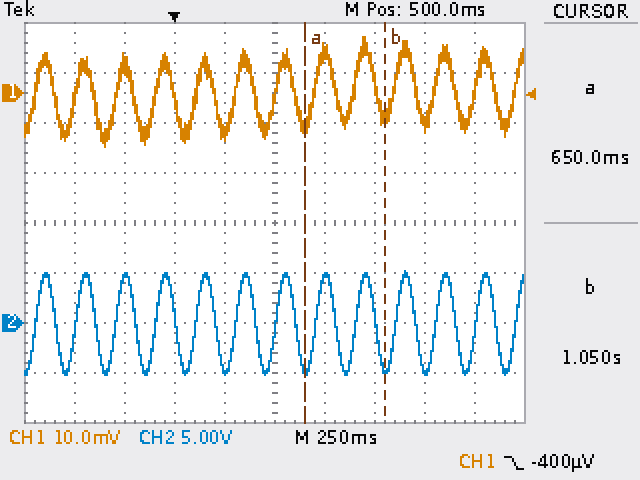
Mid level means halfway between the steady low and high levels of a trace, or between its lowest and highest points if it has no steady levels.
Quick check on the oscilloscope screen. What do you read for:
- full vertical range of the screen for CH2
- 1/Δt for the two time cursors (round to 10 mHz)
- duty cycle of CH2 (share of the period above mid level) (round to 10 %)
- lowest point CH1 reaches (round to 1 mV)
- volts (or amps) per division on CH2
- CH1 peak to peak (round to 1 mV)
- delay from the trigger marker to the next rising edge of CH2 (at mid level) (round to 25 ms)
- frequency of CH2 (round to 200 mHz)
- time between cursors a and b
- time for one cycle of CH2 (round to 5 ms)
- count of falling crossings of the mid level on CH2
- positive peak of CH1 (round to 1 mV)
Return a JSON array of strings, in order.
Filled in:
["40 V", "2.50 Hz", "50 %", "-11 mV", "5 V", "22 mV", "100 ms", "5.0 Hz", "400 ms", "200 ms", "12", "11 mV"]
